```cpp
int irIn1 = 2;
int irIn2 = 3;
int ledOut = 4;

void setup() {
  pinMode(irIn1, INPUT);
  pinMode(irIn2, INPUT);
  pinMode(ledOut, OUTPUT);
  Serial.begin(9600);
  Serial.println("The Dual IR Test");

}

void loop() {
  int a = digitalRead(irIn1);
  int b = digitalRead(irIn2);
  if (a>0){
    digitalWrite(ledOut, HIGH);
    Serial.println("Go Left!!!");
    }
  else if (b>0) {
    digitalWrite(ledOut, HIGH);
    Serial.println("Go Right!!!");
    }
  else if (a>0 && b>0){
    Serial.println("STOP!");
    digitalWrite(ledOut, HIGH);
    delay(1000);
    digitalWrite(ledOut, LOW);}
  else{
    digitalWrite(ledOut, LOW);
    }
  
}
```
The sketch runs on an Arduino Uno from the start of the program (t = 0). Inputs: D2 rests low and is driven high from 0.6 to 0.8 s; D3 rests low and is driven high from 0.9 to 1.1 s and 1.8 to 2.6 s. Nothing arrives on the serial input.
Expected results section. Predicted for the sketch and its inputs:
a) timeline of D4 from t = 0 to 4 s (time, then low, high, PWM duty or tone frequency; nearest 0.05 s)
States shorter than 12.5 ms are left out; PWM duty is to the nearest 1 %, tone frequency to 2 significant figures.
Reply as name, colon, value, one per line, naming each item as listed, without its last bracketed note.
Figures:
timeline of D4 from t = 0 to 4 s: 0 s low; 0.6 s high; 0.8 s low; 0.9 s high; 1.1 s low; 1.8 s high; 2.6 s low
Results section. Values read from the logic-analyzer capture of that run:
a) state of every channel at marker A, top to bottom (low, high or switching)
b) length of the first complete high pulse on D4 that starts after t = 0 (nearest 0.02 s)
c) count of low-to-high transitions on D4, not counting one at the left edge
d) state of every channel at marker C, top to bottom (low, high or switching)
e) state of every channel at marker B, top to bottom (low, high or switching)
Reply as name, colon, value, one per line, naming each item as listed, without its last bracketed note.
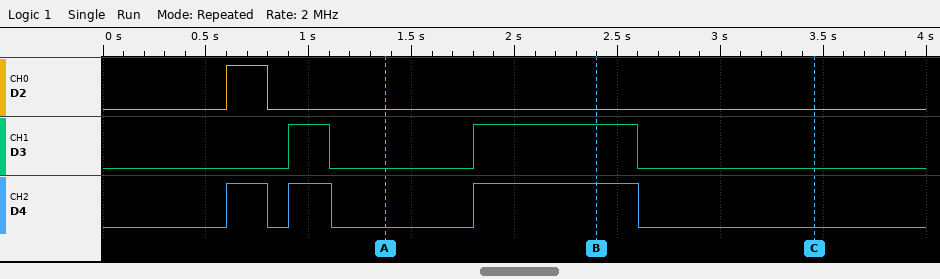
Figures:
state of every channel at marker A, top to bottom: D2 low, D3 low, D4 low
length of the first complete high pulse on D4 that starts after t = 0: 0.20 s
count of low-to-high transitions on D4, not counting one at the left edge: 3
state of every channel at marker C, top to bottom: D2 low, D3 low, D4 low
state of every channel at marker B, top to bottom: D2 low, D3 high, D4 high
